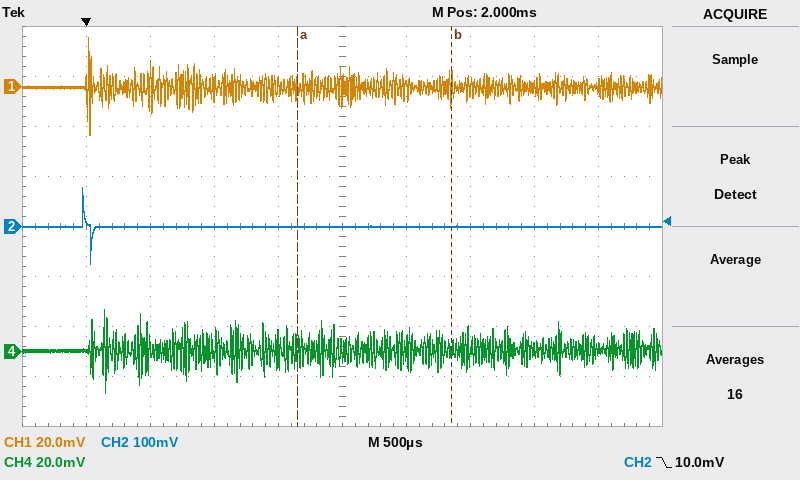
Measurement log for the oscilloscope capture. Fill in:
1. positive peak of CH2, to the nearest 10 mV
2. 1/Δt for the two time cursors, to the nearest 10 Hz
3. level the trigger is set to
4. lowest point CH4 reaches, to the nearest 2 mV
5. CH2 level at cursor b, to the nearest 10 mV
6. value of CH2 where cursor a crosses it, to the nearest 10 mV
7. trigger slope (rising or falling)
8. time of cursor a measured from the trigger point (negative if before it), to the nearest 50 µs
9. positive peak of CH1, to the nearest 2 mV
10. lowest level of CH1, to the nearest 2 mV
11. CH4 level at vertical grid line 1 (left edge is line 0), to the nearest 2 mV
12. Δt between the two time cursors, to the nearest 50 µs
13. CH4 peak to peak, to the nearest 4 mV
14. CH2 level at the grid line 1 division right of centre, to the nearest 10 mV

80 mV
830 Hz
10.0 mV
-16 mV
0 mV
0 mV
falling
+1.65 ms
20 mV
-20 mV
0 mV
1.20 ms
32 mV
0 mV
